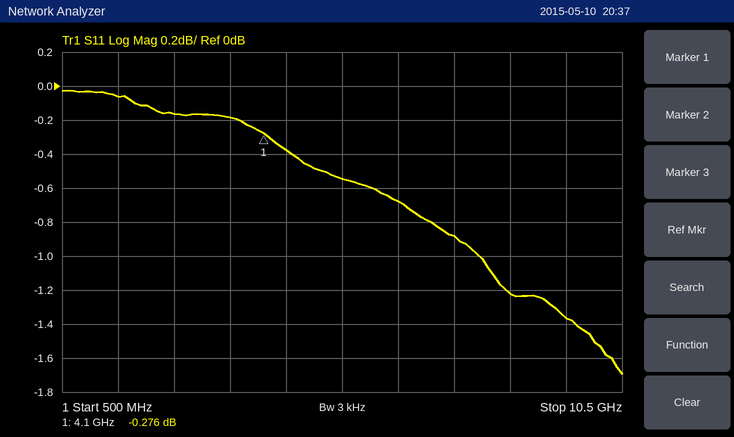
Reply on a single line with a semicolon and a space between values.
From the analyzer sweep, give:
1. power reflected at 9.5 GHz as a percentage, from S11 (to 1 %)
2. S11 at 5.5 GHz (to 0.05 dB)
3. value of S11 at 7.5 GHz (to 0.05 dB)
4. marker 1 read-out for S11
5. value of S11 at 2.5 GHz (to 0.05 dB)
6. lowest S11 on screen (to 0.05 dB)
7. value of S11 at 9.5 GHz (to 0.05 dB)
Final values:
73 %; -0.55 dB; -0.90 dB; -0.276 dB; -0.15 dB; -1.70 dB; -1.35 dB
